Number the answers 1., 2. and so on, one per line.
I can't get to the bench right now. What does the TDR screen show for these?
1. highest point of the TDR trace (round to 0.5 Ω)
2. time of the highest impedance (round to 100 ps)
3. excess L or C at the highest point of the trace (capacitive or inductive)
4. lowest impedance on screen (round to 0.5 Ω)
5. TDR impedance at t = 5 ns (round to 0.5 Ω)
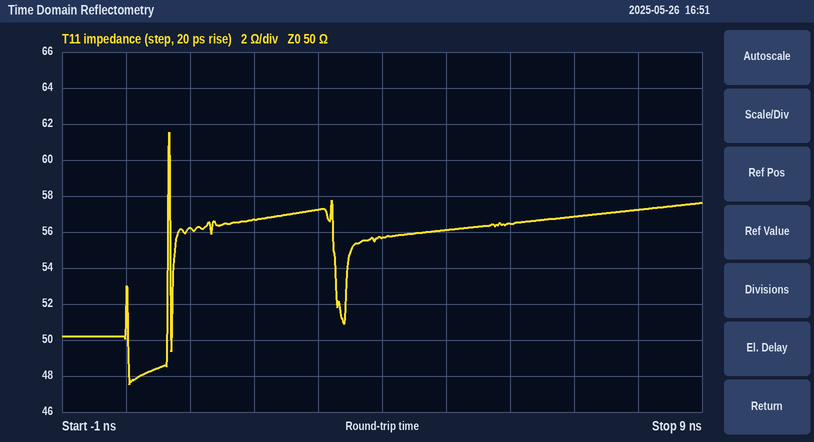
1. 61.5 Ω
2. 700 ps
3. inductive
4. 47.5 Ω
5. 56.0 Ω
